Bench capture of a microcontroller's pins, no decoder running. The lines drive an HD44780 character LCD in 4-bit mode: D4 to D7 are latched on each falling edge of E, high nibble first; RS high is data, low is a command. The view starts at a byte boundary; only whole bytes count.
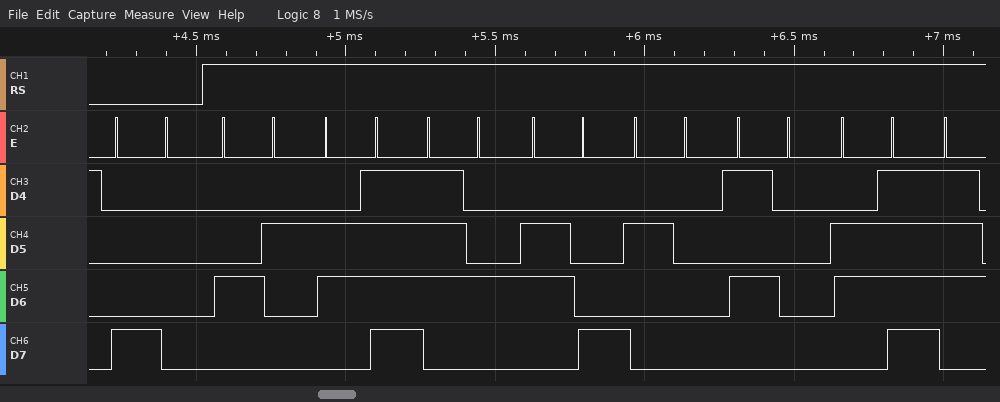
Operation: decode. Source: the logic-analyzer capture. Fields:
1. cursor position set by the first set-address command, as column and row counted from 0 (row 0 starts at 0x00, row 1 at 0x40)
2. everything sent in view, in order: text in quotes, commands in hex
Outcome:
column 0, row 0
0x80 "Both Po"
